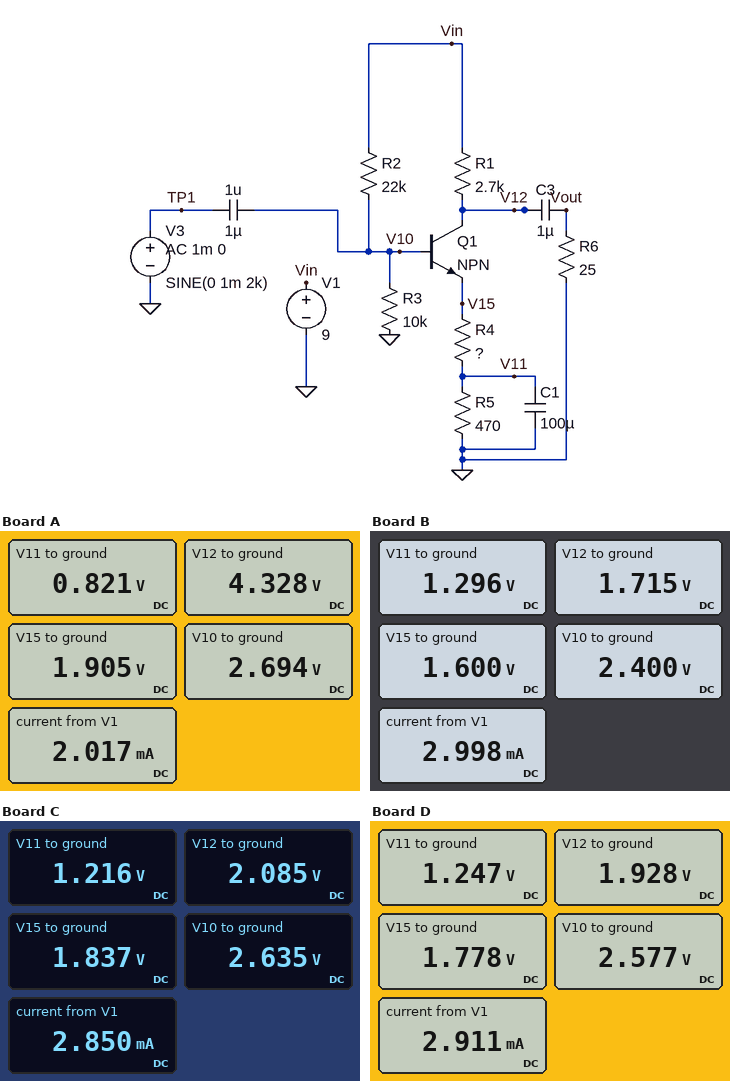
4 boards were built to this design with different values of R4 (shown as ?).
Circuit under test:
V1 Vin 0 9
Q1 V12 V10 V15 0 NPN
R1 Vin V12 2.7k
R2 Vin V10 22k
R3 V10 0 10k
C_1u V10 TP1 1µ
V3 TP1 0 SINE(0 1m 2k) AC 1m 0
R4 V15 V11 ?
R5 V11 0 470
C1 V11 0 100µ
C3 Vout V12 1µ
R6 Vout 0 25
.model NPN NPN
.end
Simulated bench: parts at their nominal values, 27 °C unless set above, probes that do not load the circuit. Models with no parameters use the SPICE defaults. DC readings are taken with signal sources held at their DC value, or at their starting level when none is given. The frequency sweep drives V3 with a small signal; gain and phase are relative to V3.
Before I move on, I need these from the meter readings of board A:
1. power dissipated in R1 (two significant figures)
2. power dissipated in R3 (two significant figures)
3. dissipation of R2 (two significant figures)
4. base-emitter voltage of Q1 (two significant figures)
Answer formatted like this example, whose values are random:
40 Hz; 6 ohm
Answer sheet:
8.1 mW; 730 µW; 1.8 mW; 790 mV
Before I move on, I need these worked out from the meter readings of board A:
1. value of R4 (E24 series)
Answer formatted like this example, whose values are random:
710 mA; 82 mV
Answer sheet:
620 Ω
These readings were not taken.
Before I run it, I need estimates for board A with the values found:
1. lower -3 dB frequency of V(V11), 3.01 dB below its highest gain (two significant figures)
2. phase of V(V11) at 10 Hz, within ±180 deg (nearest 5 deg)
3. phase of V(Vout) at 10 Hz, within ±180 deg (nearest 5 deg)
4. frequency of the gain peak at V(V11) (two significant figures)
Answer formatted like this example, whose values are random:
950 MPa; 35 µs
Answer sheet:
4.1 Hz; 10 deg; -20 deg; 12 Hz
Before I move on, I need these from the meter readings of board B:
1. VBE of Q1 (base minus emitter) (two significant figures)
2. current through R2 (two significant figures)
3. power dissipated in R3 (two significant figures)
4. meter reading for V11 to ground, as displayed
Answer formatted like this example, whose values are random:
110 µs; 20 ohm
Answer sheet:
800 mV; 300 µA; 580 µW; 1.296 V
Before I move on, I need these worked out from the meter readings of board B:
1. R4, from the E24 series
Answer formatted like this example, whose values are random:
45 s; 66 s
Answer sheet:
110 Ω
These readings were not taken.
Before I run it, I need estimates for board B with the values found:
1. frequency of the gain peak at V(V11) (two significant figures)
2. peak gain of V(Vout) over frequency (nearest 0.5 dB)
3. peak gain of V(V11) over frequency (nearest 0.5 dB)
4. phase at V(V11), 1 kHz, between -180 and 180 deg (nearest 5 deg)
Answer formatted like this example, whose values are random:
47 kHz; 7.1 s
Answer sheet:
500 Hz; -14.5 dB; -31.5 dB; -65 deg
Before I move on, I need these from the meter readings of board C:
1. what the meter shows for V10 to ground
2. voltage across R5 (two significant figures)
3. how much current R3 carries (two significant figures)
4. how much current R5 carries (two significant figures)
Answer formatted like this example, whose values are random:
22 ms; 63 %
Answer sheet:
2.635 V; 1.2 V; 260 µA; 2.6 mA
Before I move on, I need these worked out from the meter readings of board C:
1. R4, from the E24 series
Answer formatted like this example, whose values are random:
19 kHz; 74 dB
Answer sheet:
240 Ω
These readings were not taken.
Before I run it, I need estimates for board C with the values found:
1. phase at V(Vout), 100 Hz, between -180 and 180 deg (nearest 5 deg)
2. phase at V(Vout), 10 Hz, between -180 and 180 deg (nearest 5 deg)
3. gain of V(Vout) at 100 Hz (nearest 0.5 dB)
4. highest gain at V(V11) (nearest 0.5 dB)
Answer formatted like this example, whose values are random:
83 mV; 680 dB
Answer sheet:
-125 deg; -5 deg; -21.5 dB; -18.0 dB
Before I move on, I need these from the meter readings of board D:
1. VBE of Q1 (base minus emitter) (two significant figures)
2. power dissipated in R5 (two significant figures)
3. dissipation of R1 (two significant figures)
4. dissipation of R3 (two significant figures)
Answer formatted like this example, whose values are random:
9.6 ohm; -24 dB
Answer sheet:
800 mV; 3.3 mW; 19 mW; 660 µW
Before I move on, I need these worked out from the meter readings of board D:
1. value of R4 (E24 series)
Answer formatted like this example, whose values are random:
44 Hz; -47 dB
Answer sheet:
200 Ω
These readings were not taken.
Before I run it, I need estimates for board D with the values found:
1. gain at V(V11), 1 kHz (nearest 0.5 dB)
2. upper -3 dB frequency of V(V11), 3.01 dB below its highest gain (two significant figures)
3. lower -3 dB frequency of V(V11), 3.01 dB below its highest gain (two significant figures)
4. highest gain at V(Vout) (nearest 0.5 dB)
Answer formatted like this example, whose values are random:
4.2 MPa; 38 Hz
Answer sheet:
-42.0 dB; 310 Hz; 110 Hz; -18.0 dB
